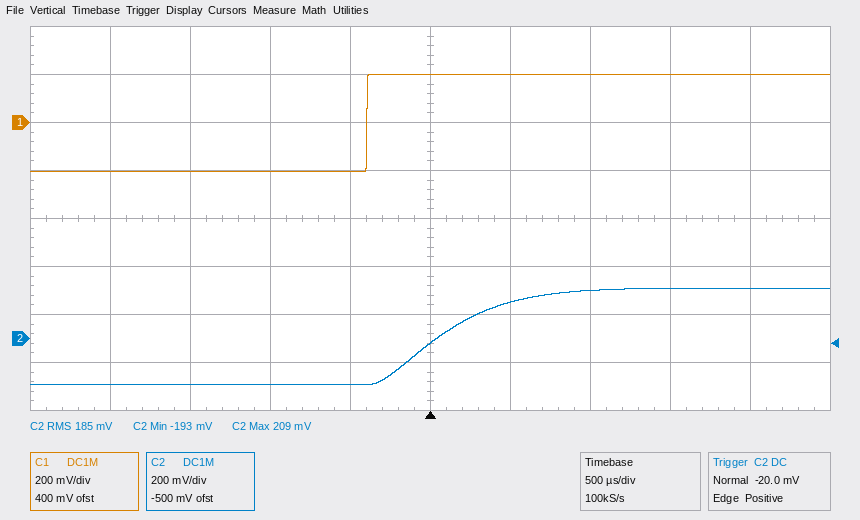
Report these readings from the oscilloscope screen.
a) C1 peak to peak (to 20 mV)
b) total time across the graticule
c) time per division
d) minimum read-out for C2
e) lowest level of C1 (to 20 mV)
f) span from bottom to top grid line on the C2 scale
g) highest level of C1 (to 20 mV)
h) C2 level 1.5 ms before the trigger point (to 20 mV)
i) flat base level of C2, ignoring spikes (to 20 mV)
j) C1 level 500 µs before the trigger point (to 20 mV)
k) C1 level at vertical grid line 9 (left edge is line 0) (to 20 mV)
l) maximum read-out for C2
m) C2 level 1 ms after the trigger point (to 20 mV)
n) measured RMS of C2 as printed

400 mV
5 ms
500 µs
-193 mV
-200 mV
1.6 V
200 mV
-200 mV
-200 mV
-200 mV
200 mV
209 mV
200 mV
185 mV
